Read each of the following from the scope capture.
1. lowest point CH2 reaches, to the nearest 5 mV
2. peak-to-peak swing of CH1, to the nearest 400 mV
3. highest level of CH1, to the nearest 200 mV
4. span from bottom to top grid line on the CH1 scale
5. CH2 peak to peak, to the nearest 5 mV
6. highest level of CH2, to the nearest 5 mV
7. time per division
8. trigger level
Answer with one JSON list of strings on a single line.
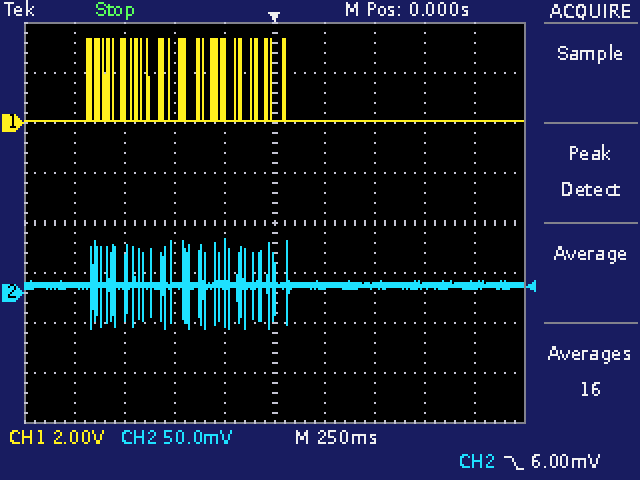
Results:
["-35 mV", "3.2 V", "3.4 V", "16 V", "90 mV", "55 mV", "250 ms", "6.00 mV"]
